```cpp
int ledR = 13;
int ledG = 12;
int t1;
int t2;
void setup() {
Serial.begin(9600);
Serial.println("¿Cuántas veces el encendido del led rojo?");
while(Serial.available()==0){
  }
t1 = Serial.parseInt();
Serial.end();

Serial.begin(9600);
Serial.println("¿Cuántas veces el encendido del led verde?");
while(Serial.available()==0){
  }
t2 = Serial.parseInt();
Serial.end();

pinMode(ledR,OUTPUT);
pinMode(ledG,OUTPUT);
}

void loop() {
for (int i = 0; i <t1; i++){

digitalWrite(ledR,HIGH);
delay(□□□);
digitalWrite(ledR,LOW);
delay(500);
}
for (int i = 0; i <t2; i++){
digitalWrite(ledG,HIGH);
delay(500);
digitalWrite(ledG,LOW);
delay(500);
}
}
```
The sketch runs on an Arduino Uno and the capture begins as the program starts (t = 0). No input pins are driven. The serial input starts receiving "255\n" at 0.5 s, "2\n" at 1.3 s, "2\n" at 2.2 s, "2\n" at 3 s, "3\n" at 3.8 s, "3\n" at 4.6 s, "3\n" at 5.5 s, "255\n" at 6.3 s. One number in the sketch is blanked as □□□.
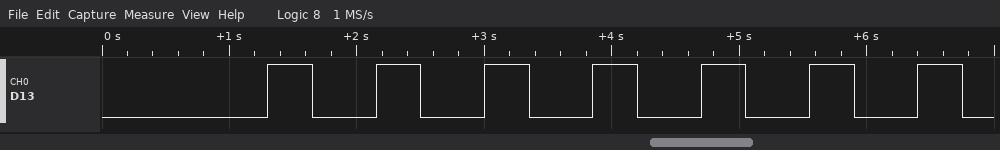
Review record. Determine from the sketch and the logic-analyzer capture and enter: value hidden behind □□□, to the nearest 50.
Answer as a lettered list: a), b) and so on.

a) 350
